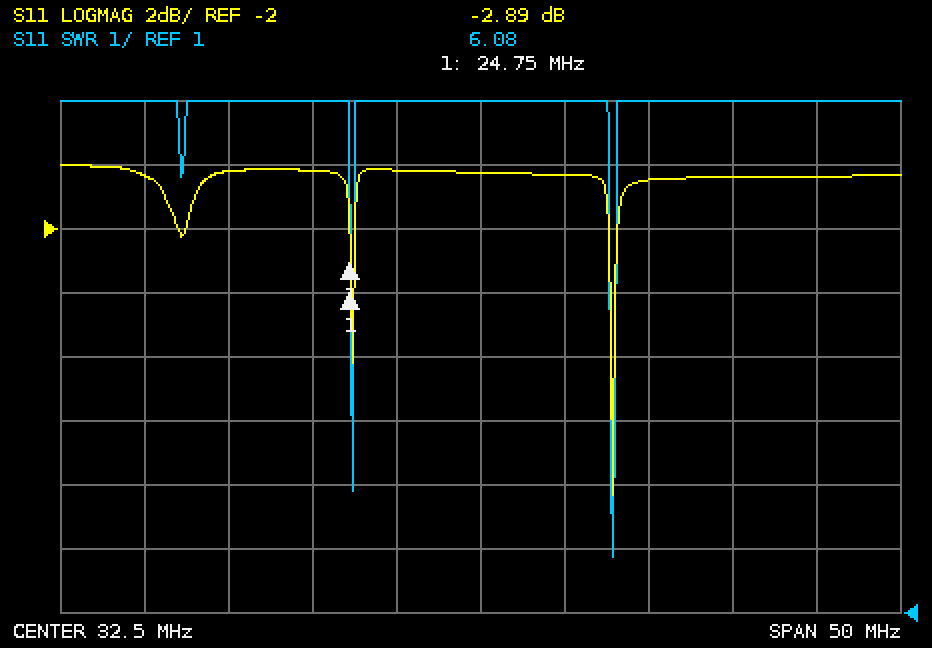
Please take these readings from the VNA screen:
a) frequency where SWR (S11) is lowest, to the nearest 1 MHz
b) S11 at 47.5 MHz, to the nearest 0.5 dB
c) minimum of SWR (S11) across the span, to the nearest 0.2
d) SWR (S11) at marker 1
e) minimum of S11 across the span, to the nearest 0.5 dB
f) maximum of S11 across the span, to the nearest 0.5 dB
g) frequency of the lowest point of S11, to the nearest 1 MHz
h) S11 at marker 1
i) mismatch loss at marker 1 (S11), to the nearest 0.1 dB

40 MHz
-0.5 dB
1.8
6.08
-10.5 dB
0.0 dB
40 MHz
-2.89 dB
3.1 dB
